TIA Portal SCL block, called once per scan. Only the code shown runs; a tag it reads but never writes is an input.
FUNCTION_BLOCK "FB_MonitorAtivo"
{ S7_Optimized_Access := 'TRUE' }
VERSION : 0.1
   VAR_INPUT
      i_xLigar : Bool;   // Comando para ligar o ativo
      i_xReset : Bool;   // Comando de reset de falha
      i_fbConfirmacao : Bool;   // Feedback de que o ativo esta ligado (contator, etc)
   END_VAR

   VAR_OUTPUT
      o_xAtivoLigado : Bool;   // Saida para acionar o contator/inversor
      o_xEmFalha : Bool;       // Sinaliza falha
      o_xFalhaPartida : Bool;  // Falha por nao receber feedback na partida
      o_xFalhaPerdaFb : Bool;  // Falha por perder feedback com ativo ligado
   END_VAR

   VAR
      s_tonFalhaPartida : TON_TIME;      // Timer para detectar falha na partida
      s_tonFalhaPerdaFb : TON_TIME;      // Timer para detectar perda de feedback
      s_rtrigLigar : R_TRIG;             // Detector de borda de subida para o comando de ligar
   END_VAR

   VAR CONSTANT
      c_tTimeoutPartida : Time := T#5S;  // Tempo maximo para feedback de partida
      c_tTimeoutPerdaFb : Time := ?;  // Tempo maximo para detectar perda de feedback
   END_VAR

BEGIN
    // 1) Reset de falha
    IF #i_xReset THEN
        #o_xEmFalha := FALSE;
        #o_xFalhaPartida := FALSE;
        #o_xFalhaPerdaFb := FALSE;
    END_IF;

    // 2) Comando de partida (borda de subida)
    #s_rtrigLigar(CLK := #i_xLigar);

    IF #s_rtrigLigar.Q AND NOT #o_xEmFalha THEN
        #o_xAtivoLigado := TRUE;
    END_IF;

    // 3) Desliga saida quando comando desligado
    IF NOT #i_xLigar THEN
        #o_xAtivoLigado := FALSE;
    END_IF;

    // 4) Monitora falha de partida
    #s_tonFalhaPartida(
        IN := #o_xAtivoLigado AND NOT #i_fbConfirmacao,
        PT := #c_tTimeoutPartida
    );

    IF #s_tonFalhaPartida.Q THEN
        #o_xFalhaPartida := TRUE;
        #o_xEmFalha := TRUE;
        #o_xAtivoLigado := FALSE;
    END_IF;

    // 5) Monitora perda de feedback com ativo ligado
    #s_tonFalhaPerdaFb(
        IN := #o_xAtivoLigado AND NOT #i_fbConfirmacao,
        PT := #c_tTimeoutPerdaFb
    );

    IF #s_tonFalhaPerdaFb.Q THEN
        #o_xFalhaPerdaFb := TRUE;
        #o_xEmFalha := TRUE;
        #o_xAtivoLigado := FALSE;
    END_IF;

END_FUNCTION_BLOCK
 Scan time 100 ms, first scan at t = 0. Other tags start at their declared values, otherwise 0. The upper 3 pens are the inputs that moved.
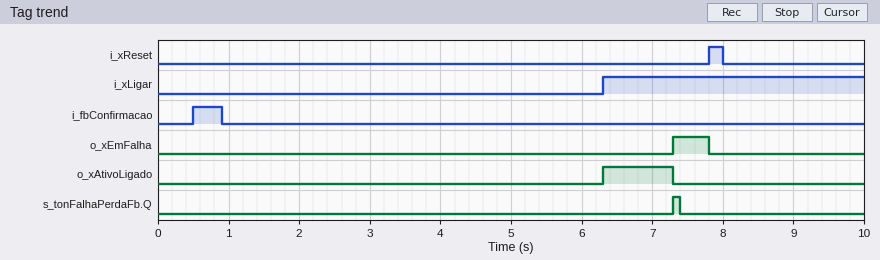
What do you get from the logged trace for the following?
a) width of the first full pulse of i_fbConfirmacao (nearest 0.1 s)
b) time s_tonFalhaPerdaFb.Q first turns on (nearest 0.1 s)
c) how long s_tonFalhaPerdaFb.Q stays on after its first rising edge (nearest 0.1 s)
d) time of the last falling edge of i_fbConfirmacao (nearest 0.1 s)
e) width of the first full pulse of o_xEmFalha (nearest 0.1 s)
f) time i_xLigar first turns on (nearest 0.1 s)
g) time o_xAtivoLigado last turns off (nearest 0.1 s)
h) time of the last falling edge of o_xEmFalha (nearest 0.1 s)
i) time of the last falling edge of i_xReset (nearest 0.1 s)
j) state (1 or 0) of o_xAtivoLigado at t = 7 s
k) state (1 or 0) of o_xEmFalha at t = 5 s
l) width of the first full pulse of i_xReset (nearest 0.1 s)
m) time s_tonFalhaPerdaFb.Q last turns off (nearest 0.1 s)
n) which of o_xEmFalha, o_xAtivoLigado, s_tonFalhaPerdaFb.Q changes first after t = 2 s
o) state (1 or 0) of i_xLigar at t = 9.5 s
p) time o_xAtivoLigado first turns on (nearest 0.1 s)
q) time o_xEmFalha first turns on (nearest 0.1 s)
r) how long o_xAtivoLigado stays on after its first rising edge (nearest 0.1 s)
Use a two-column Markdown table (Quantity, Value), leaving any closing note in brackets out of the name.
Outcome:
| Quantity | Value |
|---|---|
| width of the first full pulse of i_fbConfirmacao | 0.4 s |
| time s_tonFalhaPerdaFb.Q first turns on | 7.3 s |
| how long s_tonFalhaPerdaFb.Q stays on after its first rising edge | 0.1 s |
| time of the last falling edge of i_fbConfirmacao | 0.9 s |
| width of the first full pulse of o_xEmFalha | 0.5 s |
| time i_xLigar first turns on | 6.3 s |
| time o_xAtivoLigado last turns off | 7.3 s |
| time of the last falling edge of o_xEmFalha | 7.8 s |
| time of the last falling edge of i_xReset | 8.0 s |
| state (1 or 0) of o_xAtivoLigado at t = 7 s | 1 |
| state (1 or 0) of o_xEmFalha at t = 5 s | 0 |
| width of the first full pulse of i_xReset | 0.2 s |
| time s_tonFalhaPerdaFb.Q last turns off | 7.4 s |
| which of o_xEmFalha, o_xAtivoLigado, s_tonFalhaPerdaFb.Q changes first after t = 2 s | o_xAtivoLigado |
| state (1 or 0) of i_xLigar at t = 9.5 s | 1 |
| time o_xAtivoLigado first turns on | 6.3 s |
| time o_xEmFalha first turns on | 7.3 s |
| how long o_xAtivoLigado stays on after its first rising edge | 1.0 s |
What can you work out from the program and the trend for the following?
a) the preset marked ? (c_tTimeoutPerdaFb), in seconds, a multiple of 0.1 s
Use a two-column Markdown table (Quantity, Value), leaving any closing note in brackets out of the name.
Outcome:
| Quantity | Value |
|---|---|
| the preset marked ? (c_tTimeoutPerdaFb), in seconds, a multiple of 0.1 s | 1.0 s |
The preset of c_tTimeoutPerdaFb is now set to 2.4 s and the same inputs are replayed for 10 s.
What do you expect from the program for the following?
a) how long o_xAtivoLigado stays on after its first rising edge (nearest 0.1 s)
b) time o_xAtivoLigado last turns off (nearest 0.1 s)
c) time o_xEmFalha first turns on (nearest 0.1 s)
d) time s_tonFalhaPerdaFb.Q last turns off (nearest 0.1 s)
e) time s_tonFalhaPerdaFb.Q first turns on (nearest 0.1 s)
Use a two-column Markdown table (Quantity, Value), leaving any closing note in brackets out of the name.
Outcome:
| Quantity | Value |
|---|---|
| how long o_xAtivoLigado stays on after its first rising edge | 2.4 s |
| time o_xAtivoLigado last turns off | 8.7 s |
| time o_xEmFalha first turns on | 8.7 s |
| time s_tonFalhaPerdaFb.Q last turns off | 8.8 s |
| time s_tonFalhaPerdaFb.Q first turns on | 8.7 s |
